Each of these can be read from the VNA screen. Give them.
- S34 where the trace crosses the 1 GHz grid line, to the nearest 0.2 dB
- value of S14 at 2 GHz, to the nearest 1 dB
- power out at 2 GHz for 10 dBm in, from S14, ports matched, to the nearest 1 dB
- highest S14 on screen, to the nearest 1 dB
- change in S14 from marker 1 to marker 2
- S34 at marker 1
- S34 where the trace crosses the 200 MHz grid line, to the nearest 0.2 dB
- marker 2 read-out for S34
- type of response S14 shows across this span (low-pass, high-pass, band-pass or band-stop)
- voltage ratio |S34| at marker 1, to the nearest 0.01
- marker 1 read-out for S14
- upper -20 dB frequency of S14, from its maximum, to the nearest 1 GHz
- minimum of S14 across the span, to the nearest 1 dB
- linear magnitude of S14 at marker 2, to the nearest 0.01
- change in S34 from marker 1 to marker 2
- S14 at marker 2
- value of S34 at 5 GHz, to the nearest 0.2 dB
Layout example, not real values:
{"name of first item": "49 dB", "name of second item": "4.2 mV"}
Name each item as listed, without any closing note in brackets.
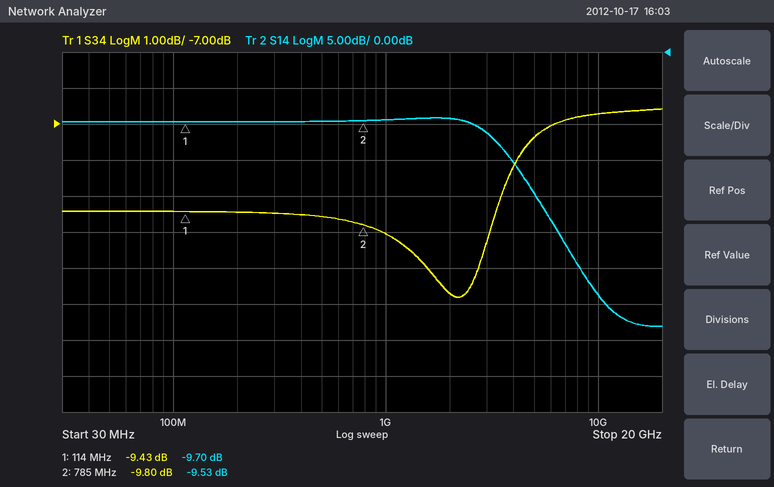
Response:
{"S34 where the trace crosses the 1 GHz grid line, to the nearest 0.2 dB": "-10.0 dB", "value of S14 at 2 GHz, to the nearest 1 dB": "-9 dB", "power out at 2 GHz for 10 dBm in, from S14, ports matched, to the nearest 1 dB": "1 dBm", "highest S14 on screen, to the nearest 1 dB": "-9 dB", "change in S14 from marker 1 to marker 2": "0.17 dB", "S34 at marker 1": "-9.43 dB", "S34 where the trace crosses the 200 MHz grid line, to the nearest 0.2 dB": "-9.4 dB", "marker 2 read-out for S34": "-9.80 dB", "type of response S14 shows across this span": "low-pass", "voltage ratio |S34| at marker 1, to the nearest 0.01": "0.34", "marker 1 read-out for S14": "-9.70 dB", "upper -20 dB frequency of S14, from its maximum, to the nearest 1 GHz": "8 GHz", "minimum of S14 across the span, to the nearest 1 dB": "-38 dB", "linear magnitude of S14 at marker 2, to the nearest 0.01": "0.33", "change in S34 from marker 1 to marker 2": "-0.37 dB", "S14 at marker 2": "-9.53 dB", "value of S34 at 5 GHz, to the nearest 0.2 dB": "-7.4 dB"}
